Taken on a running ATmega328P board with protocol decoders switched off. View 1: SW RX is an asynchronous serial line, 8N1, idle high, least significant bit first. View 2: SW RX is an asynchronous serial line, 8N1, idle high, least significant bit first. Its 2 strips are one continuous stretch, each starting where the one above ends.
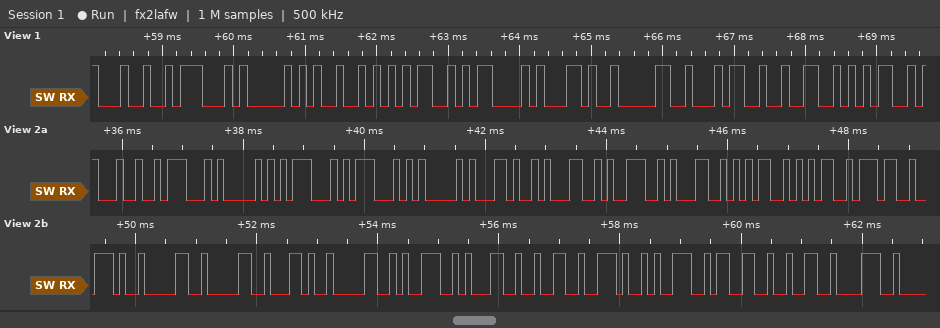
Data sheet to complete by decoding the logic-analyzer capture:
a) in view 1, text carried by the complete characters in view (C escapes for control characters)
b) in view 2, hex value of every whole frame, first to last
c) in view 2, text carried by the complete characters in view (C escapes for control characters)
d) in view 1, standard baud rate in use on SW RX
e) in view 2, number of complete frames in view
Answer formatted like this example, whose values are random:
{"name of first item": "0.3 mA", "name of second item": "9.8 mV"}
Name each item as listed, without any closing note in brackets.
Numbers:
{"in view 1, text carried by the complete characters in view": "\"$GPRMC,0425\"", "in view 2, hex value of every whole frame, first to last": "24 47 50 47 47 41 2C 31 39 31 35 35 37 2E 30 30 2C 30 39 31 32 2E 39 33 32 38", "in view 2, text carried by the complete characters in view": "\"$GPGGA,191557.00,0912.9328\"", "in view 1, standard baud rate in use on SW RX": "9600 baud", "in view 2, number of complete frames in view": "26"}
